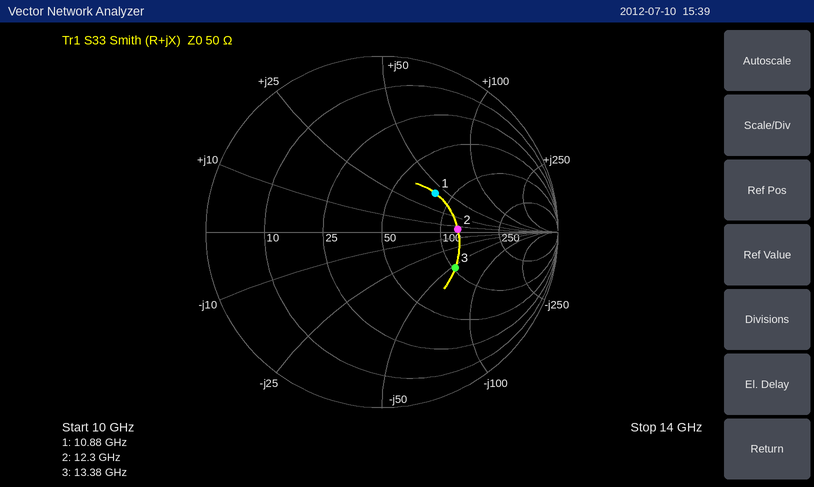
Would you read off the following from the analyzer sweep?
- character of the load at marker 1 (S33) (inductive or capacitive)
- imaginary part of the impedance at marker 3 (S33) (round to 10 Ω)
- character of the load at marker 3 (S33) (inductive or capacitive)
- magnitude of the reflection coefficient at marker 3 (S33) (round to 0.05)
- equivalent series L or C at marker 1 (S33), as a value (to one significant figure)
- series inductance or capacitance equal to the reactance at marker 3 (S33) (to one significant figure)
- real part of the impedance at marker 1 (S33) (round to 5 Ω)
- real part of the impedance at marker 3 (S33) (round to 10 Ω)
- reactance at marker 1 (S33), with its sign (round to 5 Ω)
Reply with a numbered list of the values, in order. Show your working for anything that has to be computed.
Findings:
1. inductive
2. -50 Ω
3. capacitive
4. 0.45
5. L = 40 Ω/(2π × 10.88 GHz) ≈ 585 pH, so 600 pH to one significant figure
6. C = 1/(2π × 13.38 GHz × 50 Ω) ≈ 238 fF, so 200 fF to one significant figure
7. 80 Ω
8. 100 Ω
9. +40 Ω
